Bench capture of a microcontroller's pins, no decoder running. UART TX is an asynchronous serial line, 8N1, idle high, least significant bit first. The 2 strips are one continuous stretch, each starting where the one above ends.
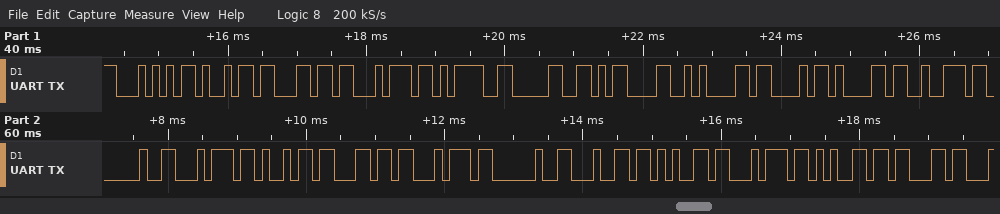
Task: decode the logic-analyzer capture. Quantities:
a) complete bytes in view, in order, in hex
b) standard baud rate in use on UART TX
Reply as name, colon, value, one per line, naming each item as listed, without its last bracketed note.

complete bytes in view, in order, in hex: 0x54 0x69 0x6C 0x74 0x3D 0x30 0x0D 0x0A 0x43 0x61 0x72 0x20 0x74 0x69 0x6C 0x74 0x20 0x64 0x65 0x74 0x65 0x63
standard baud rate in use on UART TX: 9600 baud
